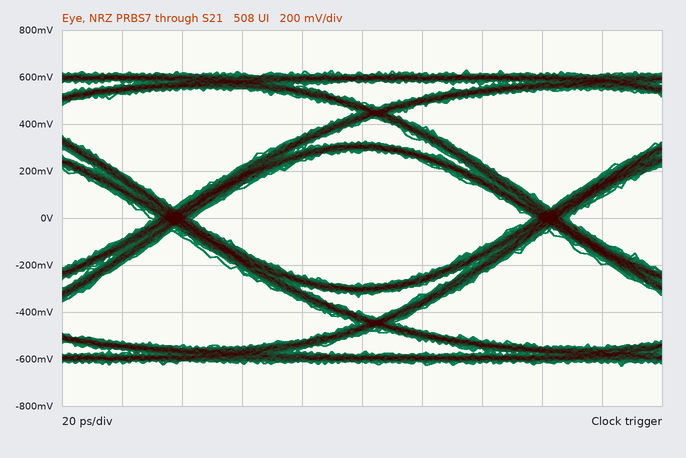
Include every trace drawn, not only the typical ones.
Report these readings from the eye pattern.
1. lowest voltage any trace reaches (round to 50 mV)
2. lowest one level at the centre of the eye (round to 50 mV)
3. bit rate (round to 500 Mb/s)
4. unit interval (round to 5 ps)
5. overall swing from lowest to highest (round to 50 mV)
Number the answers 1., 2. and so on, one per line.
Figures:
1. -650 mV
2. 300 mV
3. 8.0 Gb/s
4. 125 ps
5. 1.25 V
